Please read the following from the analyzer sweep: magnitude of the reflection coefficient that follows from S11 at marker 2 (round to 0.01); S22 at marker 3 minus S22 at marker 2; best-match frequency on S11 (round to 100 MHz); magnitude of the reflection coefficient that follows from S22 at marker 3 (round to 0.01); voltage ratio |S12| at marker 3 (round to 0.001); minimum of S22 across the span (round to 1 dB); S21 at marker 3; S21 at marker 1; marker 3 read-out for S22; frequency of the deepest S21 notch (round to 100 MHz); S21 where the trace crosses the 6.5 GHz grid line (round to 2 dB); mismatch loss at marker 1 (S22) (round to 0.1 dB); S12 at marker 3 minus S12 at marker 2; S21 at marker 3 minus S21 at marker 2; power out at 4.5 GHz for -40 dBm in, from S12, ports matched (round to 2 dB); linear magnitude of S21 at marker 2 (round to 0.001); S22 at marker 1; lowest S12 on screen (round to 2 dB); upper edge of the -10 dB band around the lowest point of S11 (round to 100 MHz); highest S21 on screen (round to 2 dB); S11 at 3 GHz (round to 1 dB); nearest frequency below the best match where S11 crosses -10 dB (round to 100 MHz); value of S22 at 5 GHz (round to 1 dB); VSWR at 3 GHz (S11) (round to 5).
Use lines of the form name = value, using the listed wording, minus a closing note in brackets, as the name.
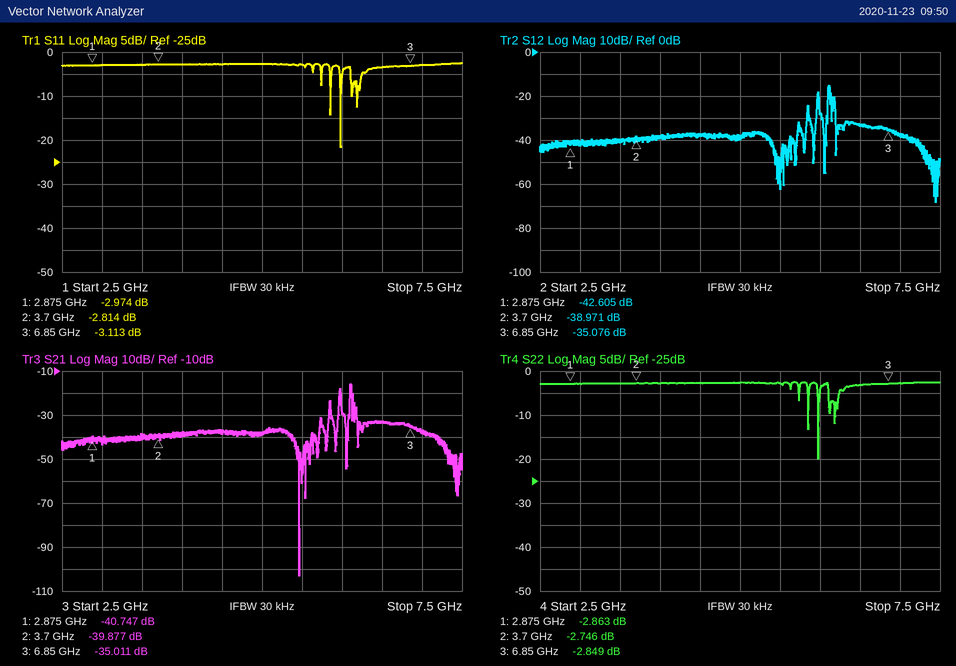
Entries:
magnitude of the reflection coefficient that follows from S11 at marker 2 = 0.72
S22 at marker 3 minus S22 at marker 2 = -0.103 dB
best-match frequency on S11 = 6.0 GHz
magnitude of the reflection coefficient that follows from S22 at marker 3 = 0.72
voltage ratio |S12| at marker 3 = 0.018
minimum of S22 across the span = -20 dB
S21 at marker 3 = -35.011 dB
S21 at marker 1 = -40.747 dB
marker 3 read-out for S22 = -2.849 dB
frequency of the deepest S21 notch = 5.5 GHz
S21 where the trace crosses the 6.5 GHz grid line = -34 dB
mismatch loss at marker 1 (S22) = 3.2 dB
S12 at marker 3 minus S12 at marker 2 = 3.895 dB
S21 at marker 3 minus S21 at marker 2 = 4.866 dB
power out at 4.5 GHz for -40 dBm in, from S12, ports matched = -78 dBm
linear magnitude of S21 at marker 2 = 0.010
S22 at marker 1 = -2.863 dB
lowest S12 on screen = -68 dB
upper edge of the -10 dB band around the lowest point of S11 = 6.0 GHz
highest S21 on screen = -16 dB
S11 at 3 GHz = -3 dB
nearest frequency below the best match where S11 crosses -10 dB = 6.0 GHz
value of S22 at 5 GHz = -3 dB
VSWR at 3 GHz (S11) = 5
